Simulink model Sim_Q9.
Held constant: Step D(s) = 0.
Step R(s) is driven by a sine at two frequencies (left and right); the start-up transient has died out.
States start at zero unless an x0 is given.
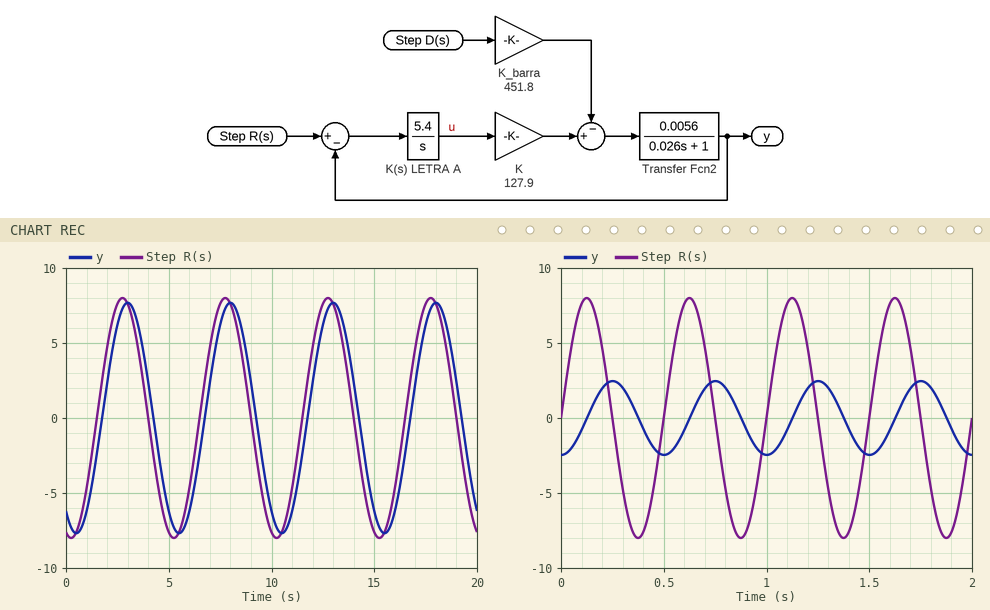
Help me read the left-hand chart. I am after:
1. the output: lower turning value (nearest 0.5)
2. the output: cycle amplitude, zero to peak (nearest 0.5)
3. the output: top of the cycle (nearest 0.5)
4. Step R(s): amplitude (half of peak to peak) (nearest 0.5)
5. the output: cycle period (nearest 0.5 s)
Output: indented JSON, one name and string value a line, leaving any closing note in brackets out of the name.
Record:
{
  "the output: lower turning value": "-7.5",
  "the output: cycle amplitude, zero to peak": "7.5",
  "the output: top of the cycle": "7.5",
  "Step R(s): amplitude (half of peak to peak)": "8.0",
  "the output: cycle period": "5.0 s"
}
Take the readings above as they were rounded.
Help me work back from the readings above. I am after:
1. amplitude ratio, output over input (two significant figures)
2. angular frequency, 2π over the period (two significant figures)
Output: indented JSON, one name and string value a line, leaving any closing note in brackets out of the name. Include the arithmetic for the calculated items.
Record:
{
  "amplitude ratio, output over input": "7.5 / 8 = 0.94",
  "angular frequency, 2π over the period": "2π / 5 = 1.3 rad/s"
}
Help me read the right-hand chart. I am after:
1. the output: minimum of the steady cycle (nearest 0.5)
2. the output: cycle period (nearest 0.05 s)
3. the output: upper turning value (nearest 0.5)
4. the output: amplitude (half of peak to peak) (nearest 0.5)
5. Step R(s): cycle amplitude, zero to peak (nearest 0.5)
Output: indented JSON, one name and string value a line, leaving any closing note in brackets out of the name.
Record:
{
  "the output: minimum of the steady cycle": "-2.5",
  "the output: cycle period": "0.50 s",
  "the output: upper turning value": "2.5",
  "the output: amplitude (half of peak to peak)": "2.5",
  "Step R(s): cycle amplitude, zero to peak": "8.0"
}
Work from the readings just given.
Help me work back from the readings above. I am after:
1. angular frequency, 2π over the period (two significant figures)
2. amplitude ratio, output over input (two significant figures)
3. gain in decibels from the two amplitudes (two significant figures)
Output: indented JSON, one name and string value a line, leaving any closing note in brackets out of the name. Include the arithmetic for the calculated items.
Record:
{
  "angular frequency, 2π over the period": "2π / 0.5 = 13 rad/s",
  "amplitude ratio, output over input": "2.5 / 8 = 0.31",
  "gain in decibels from the two amplitudes": "20 log10(2.5 / 8) = -10 dB"
}
